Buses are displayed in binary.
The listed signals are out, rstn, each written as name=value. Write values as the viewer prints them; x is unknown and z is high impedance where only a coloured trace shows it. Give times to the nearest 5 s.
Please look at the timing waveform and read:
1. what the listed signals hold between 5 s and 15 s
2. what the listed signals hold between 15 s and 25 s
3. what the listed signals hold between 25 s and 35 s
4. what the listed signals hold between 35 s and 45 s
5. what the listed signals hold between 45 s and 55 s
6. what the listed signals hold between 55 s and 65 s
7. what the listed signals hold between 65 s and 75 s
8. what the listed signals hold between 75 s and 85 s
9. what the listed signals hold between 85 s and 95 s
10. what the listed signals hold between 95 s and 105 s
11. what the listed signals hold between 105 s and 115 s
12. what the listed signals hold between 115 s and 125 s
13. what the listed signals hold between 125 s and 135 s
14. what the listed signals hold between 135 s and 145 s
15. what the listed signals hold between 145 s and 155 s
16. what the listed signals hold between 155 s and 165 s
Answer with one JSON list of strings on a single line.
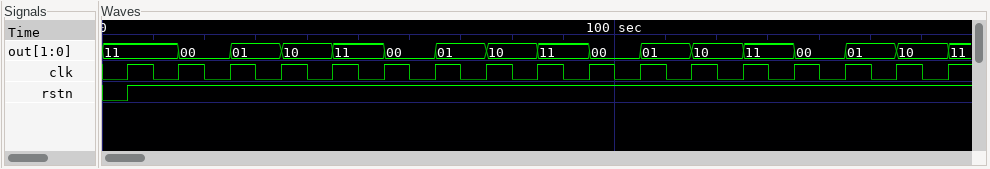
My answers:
["out=11, rstn=1", "out=00, rstn=1", "out=01, rstn=1", "out=10, rstn=1", "out=11, rstn=1", "out=00, rstn=1", "out=01, rstn=1", "out=10, rstn=1", "out=11, rstn=1", "out=00, rstn=1", "out=01, rstn=1", "out=10, rstn=1", "out=11, rstn=1", "out=00, rstn=1", "out=01, rstn=1", "out=10, rstn=1"]
